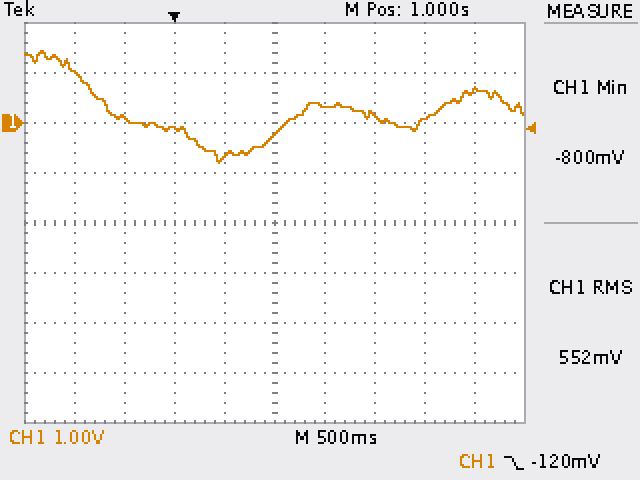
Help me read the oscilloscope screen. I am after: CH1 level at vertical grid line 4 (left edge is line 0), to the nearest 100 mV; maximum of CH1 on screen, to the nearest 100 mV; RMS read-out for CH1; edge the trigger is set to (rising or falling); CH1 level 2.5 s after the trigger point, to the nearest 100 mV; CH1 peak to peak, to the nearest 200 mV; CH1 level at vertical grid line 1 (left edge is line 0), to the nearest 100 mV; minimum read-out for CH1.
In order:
-700 mV
1.4 V
552 mV
falling
100 mV
2.2 V
1.0 V
-800 mV
